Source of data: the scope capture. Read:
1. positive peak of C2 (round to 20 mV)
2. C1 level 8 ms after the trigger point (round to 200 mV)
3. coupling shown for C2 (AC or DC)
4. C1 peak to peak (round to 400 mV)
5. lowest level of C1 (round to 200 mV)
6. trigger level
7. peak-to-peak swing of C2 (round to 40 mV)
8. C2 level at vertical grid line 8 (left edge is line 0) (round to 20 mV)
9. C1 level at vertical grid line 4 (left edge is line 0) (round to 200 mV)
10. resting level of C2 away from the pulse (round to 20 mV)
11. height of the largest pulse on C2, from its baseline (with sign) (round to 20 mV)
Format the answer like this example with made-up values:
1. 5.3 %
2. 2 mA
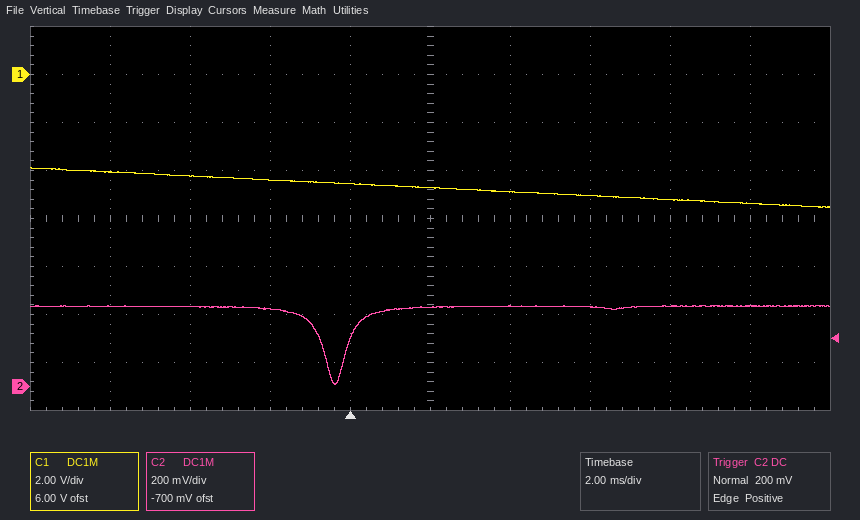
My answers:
1. 340 mV
2. -5.2 V
3. DC
4. 1.6 V
5. -5.6 V
6. 200 mV
7. 320 mV
8. 340 mV
9. -4.6 V
10. 340 mV
11. -320 mV
